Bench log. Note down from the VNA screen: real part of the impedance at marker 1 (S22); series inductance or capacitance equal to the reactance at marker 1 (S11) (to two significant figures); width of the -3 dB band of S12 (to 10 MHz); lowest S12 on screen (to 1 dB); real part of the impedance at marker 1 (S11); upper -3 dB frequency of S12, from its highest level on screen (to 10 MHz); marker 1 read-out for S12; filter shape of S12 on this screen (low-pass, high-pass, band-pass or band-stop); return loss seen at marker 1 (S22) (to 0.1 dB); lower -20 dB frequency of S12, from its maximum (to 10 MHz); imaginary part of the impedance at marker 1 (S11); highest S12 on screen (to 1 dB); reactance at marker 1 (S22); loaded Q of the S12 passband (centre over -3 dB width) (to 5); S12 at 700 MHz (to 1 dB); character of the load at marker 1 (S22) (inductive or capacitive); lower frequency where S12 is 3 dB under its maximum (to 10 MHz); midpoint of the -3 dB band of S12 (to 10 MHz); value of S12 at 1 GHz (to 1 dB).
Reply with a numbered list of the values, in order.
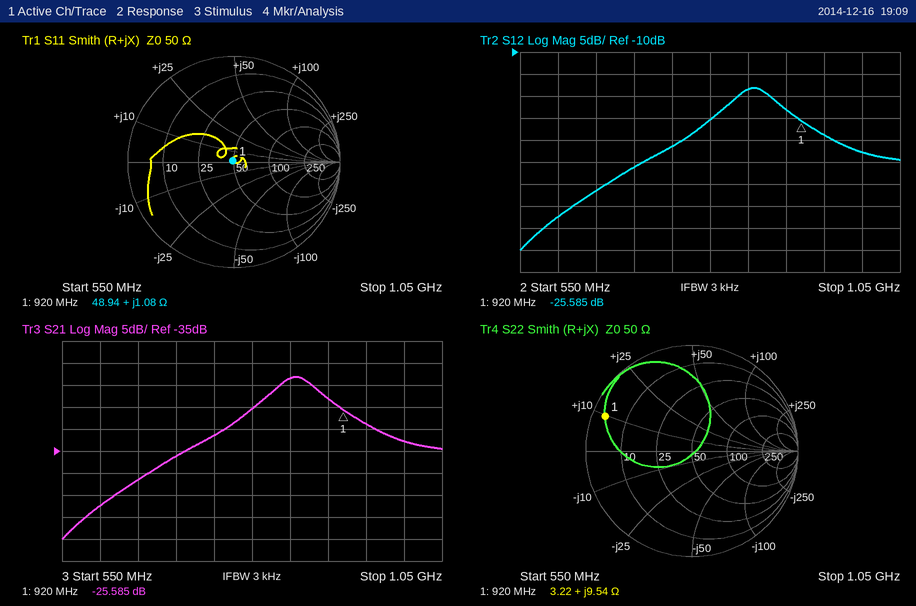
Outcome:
1. 3.22 Ω
2. 190 pH
3. 60 MHz
4. -55 dB
5. 48.94 Ω
6. 890 MHz
7. -25.585 dB
8. band-pass
9. 1.1 dB
10. 680 MHz
11. +1.08 Ω
12. -18 dB
13. +9.54 Ω
14. 15
15. -36 dB
16. inductive
17. 830 MHz
18. 860 MHz
19. -33 dB
